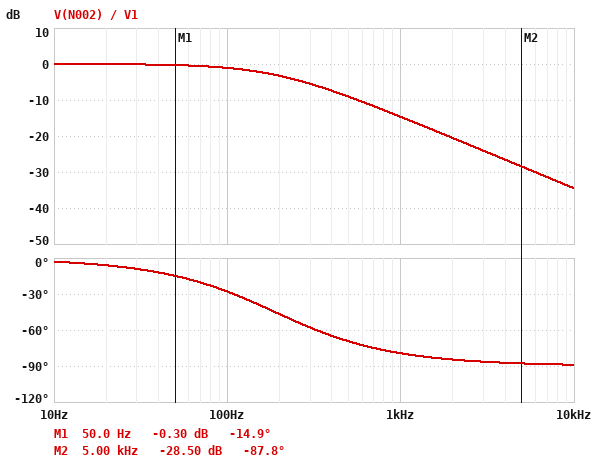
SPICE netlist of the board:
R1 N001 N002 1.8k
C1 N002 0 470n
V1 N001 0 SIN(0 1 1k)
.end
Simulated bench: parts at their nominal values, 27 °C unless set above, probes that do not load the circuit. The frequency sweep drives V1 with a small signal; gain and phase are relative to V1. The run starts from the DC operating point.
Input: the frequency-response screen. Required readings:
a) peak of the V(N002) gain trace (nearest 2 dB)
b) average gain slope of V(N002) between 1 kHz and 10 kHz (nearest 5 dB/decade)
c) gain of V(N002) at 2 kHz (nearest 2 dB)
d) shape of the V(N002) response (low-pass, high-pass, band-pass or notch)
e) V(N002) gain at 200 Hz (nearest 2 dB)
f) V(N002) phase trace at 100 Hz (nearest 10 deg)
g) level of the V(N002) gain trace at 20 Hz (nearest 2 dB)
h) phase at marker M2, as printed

0 dB
-20 dB/decade
-20 dB
low-pass
-4 dB
-30 deg
0 dB
-87.8 deg
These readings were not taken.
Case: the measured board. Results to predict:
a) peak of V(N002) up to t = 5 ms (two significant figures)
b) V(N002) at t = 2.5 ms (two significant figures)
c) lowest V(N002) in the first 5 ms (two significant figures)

290 mV
190 mV
-180 mV
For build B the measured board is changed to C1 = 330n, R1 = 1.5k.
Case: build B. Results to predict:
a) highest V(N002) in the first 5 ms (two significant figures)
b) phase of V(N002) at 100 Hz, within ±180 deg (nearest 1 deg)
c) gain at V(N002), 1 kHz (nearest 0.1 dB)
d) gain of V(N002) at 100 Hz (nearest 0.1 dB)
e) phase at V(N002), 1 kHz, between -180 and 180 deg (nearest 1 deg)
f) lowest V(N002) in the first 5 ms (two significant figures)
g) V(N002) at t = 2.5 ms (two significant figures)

430 mV
-17 deg
-10.3 dB
-0.4 dB
-72 deg
-310 mV
290 mV
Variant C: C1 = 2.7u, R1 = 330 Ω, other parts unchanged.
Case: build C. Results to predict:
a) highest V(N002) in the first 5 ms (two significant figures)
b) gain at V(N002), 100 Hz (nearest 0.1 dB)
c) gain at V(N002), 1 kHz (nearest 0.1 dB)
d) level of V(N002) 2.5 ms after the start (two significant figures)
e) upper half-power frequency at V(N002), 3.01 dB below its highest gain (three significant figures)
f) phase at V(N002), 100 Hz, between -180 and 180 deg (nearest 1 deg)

280 mV
-1.2 dB
-15.1 dB
180 mV
179 Hz
-29 deg
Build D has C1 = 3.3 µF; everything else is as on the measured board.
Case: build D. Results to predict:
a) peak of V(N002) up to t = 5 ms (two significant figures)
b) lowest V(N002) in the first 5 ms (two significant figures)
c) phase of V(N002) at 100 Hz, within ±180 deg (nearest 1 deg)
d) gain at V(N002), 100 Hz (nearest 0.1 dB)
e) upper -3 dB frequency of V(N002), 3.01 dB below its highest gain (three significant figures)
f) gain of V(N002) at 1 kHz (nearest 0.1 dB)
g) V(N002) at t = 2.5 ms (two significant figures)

51 mV
-15 mV
-75 deg
-11.7 dB
26.8 Hz
-31.4 dB
44 mV
